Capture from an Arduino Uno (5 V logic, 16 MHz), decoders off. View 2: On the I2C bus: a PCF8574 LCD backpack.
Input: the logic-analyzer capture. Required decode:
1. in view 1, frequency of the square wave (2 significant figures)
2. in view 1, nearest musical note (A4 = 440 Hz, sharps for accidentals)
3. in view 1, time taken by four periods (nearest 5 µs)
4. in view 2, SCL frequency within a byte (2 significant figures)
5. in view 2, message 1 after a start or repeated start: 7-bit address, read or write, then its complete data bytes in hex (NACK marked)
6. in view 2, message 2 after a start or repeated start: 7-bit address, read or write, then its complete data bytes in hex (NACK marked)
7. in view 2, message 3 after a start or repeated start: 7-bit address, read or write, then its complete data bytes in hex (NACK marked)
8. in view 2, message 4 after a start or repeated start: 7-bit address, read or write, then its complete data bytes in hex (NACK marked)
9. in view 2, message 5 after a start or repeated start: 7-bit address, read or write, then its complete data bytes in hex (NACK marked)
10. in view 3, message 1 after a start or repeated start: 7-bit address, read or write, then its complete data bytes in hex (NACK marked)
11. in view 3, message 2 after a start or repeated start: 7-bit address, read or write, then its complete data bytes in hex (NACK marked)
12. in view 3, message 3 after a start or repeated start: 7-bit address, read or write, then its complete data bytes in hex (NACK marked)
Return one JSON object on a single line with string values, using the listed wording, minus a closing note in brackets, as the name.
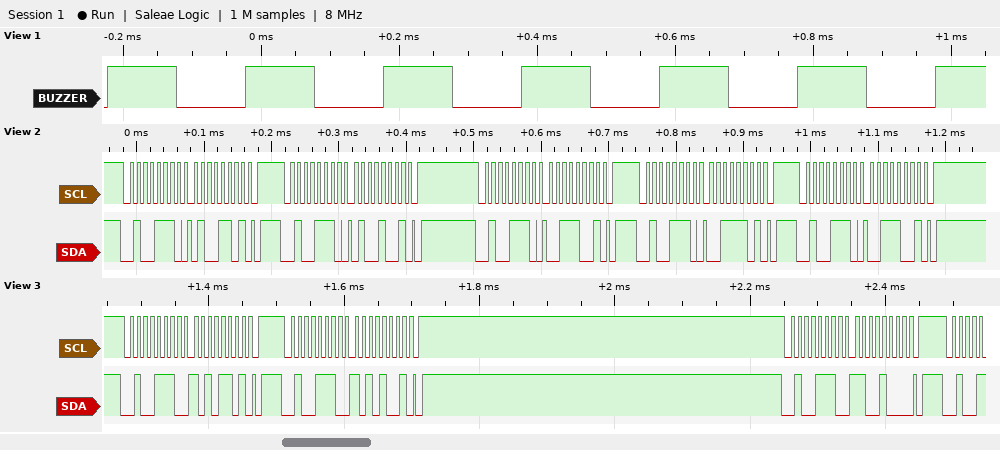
{"in view 1, frequency of the square wave": "5.0 kHz", "in view 1, nearest musical note": "D#8", "in view 1, time taken by four periods": "800 µs", "in view 2, SCL frequency within a byte": "100 kHz", "in view 2, message 1 after a start or repeated start: 7-bit address, read or write, then its complete data bytes in hex": "0x27 write: 4D", "in view 2, message 2 after a start or repeated start: 7-bit address, read or write, then its complete data bytes in hex": "0x27 write: 49", "in view 2, message 3 after a start or repeated start: 7-bit address, read or write, then its complete data bytes in hex": "0x27 write: 39", "in view 2, message 4 after a start or repeated start: 7-bit address, read or write, then its complete data bytes in hex": "0x27 write: 3D", "in view 2, message 5 after a start or repeated start: 7-bit address, read or write, then its complete data bytes in hex": "0x27 write: 39", "in view 3, message 1 after a start or repeated start: 7-bit address, read or write, then its complete data bytes in hex": "0x27 write: AD", "in view 3, message 2 after a start or repeated start: 7-bit address, read or write, then its complete data bytes in hex": "0x27 write: A9", "in view 3, message 3 after a start or repeated start: 7-bit address, read or write, then its complete data bytes in hex": "0x27 write: C8"}
